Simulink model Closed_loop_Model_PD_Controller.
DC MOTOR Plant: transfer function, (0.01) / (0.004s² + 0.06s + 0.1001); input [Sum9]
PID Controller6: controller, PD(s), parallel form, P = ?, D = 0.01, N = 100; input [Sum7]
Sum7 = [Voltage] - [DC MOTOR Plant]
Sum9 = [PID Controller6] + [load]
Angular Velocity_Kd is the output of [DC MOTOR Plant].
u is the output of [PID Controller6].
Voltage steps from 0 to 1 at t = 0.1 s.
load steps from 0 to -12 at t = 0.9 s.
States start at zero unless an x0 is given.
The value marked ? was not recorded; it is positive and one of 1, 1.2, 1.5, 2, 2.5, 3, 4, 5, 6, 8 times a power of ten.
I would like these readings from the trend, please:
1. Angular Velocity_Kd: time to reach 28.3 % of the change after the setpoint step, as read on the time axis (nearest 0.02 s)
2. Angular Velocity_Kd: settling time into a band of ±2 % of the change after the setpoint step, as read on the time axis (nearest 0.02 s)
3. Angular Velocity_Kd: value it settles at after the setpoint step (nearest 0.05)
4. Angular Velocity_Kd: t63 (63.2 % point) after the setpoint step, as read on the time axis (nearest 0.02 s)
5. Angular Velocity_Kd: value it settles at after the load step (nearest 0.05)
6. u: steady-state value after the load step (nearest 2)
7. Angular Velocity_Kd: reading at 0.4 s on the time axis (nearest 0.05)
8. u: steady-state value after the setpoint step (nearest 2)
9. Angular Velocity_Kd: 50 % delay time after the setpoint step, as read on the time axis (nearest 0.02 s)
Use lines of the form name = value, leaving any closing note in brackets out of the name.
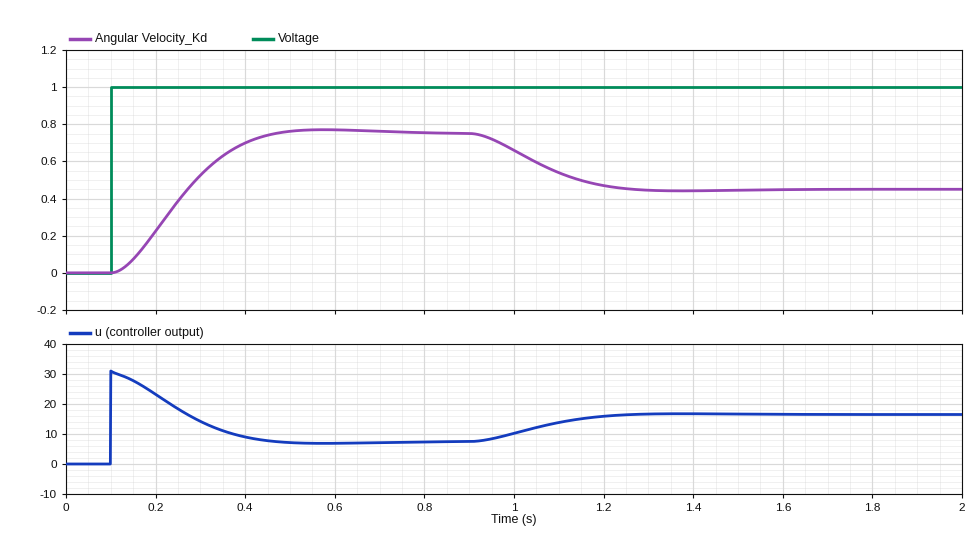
Angular Velocity_Kd: time to reach 28.3 % of the change after the setpoint step, as read on the time axis = 0.20 s
Angular Velocity_Kd: settling time into a band of ±2 % of the change after the setpoint step, as read on the time axis = 0.68 s
Angular Velocity_Kd: value it settles at after the setpoint step = 0.75
Angular Velocity_Kd: t63 (63.2 % point) after the setpoint step, as read on the time axis = 0.28 s
Angular Velocity_Kd: value it settles at after the load step = 0.45
u: steady-state value after the load step = 16
Angular Velocity_Kd: reading at 0.4 s on the time axis = 0.70
u: steady-state value after the setpoint step = 8
Angular Velocity_Kd: 50 % delay time after the setpoint step, as read on the time axis = 0.24 s
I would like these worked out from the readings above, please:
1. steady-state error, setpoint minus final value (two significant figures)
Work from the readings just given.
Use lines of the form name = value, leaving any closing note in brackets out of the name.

steady-state error, setpoint minus final value = 0.25
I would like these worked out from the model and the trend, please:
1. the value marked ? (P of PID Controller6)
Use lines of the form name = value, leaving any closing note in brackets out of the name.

the value marked ? = 30
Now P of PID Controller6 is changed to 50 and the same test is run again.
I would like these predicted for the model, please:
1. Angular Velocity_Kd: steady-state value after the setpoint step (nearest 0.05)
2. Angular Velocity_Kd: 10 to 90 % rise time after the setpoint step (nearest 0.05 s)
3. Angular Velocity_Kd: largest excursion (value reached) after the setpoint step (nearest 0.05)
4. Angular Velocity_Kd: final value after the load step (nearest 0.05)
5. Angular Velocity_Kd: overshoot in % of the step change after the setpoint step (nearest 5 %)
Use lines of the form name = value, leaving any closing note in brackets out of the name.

Angular Velocity_Kd: steady-state value after the setpoint step = 0.85
Angular Velocity_Kd: 10 to 90 % rise time after the setpoint step = 0.15 s
Angular Velocity_Kd: largest excursion (value reached) after the setpoint step = 0.90
Angular Velocity_Kd: final value after the load step = 0.65
Angular Velocity_Kd: overshoot in % of the step change after the setpoint step = 10 %
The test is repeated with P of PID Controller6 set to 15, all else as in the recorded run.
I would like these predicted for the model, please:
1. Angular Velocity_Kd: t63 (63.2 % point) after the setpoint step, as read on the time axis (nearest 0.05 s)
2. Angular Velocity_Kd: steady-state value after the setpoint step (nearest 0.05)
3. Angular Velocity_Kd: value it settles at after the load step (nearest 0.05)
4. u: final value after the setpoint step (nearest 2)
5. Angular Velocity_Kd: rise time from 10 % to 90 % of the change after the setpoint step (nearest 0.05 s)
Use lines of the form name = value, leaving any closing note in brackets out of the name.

Angular Velocity_Kd: t63 (63.2 % point) after the setpoint step, as read on the time axis = 0.35 s
Angular Velocity_Kd: steady-state value after the setpoint step = 0.60
Angular Velocity_Kd: value it settles at after the load step = 0.10
u: final value after the setpoint step = 6
Angular Velocity_Kd: rise time from 10 % to 90 % of the change after the setpoint step = 0.40 s
